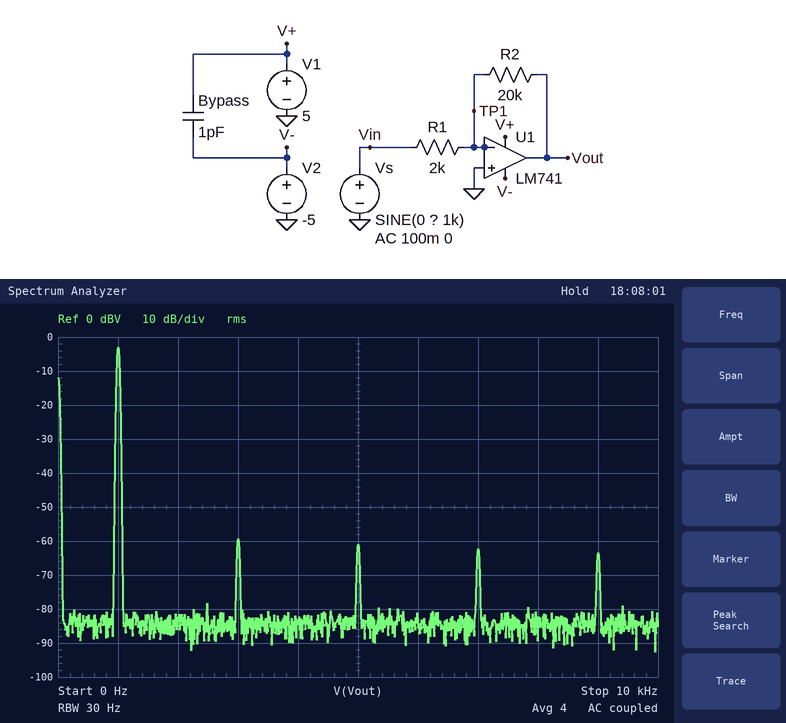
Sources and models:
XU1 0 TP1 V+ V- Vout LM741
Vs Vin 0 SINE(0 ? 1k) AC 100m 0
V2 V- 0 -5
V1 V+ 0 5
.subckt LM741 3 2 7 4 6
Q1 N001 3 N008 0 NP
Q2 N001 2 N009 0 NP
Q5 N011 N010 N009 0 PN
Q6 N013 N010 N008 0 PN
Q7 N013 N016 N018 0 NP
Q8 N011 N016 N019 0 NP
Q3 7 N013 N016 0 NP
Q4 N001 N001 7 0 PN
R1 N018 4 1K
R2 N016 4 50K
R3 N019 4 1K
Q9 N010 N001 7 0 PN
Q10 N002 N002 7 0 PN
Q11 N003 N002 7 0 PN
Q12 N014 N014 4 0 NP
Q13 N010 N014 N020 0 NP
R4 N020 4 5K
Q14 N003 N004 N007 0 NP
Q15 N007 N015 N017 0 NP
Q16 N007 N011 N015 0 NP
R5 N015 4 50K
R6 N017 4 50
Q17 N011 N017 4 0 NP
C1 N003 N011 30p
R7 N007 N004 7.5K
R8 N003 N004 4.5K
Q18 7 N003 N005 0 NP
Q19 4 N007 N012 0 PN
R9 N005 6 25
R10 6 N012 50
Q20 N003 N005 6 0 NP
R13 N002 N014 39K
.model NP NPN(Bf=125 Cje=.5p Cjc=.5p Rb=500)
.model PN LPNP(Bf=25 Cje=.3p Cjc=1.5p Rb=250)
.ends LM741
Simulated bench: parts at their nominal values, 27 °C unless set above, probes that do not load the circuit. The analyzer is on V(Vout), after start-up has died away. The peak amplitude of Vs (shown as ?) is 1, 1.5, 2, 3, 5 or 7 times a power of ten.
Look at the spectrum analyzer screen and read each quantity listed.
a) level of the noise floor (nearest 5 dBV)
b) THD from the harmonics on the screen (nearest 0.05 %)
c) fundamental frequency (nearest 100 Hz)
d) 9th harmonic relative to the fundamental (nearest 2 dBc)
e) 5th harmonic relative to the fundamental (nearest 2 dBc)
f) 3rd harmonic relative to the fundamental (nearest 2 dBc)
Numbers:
-85 dBV
0.25 %
1.0 kHz
-60 dBc
-58 dBc
-56 dBc
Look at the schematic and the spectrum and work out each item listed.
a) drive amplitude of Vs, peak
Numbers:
100 mV
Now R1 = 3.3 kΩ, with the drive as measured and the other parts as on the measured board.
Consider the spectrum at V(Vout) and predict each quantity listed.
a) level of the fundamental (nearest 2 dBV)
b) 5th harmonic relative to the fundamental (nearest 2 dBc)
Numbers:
-8 dBV
-60 dBc
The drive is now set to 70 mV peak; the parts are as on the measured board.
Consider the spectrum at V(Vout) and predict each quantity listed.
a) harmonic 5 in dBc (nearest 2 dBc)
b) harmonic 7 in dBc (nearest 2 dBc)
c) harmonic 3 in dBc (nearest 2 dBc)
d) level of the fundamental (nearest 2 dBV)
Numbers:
-56 dBc
-58 dBc
-54 dBc
-6 dBV
